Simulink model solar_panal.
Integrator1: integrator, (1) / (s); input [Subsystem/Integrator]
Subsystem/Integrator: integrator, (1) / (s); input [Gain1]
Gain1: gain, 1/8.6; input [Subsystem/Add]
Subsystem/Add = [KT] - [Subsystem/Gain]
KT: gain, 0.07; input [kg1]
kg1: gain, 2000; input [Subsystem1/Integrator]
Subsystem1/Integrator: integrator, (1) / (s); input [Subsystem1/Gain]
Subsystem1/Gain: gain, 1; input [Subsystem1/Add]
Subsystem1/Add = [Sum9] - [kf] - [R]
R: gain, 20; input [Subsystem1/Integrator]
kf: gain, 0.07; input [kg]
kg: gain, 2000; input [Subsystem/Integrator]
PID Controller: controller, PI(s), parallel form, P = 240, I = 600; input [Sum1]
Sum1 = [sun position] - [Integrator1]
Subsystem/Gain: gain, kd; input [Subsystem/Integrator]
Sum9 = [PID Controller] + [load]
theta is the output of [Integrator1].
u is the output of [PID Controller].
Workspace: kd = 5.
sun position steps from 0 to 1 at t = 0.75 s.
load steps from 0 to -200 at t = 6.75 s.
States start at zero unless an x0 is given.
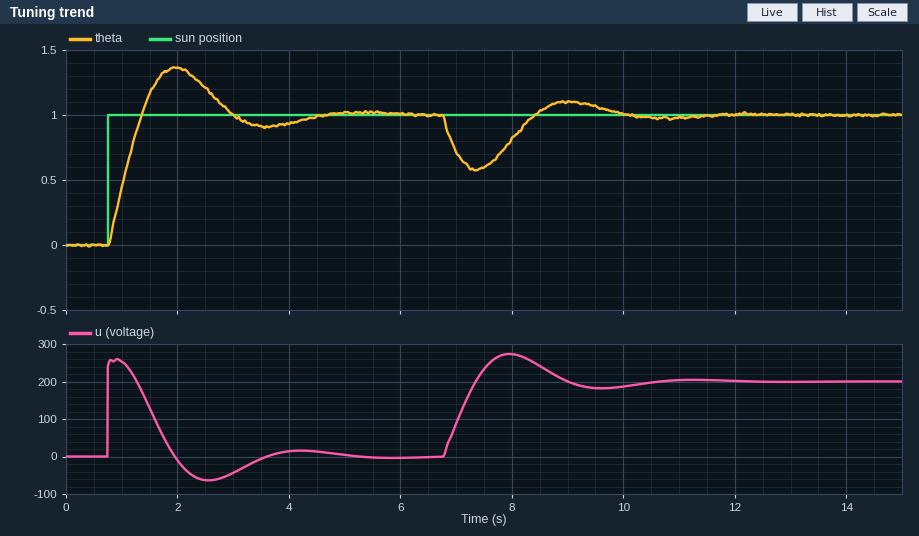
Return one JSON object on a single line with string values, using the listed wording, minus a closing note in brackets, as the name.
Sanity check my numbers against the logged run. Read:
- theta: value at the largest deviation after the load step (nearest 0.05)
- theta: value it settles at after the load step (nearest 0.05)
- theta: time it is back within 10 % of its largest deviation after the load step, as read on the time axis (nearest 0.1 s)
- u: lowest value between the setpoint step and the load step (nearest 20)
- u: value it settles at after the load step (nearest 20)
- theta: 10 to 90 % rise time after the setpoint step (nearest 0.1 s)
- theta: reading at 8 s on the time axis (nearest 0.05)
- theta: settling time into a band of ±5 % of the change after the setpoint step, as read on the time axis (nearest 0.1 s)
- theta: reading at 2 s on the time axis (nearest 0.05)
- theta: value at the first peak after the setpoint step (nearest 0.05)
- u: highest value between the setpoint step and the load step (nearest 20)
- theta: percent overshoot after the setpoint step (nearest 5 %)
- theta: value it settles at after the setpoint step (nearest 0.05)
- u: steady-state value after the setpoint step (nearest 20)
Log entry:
{"theta: value at the largest deviation after the load step": "0.60", "theta: value it settles at after the load step": "1.00", "theta: time it is back within 10 % of its largest deviation after the load step, as read on the time axis": "9.7 s", "u: lowest value between the setpoint step and the load step": "-60", "u: value it settles at after the load step": "200", "theta: 10 to 90 % rise time after the setpoint step": "0.5 s", "theta: reading at 8 s on the time axis": "0.80", "theta: settling time into a band of ±5 % of the change after the setpoint step, as read on the time axis": "4.2 s", "theta: reading at 2 s on the time axis": "1.35", "theta: value at the first peak after the setpoint step": "1.35", "u: highest value between the setpoint step and the load step": "260", "theta: percent overshoot after the setpoint step": "35 %", "theta: value it settles at after the setpoint step": "1.00", "u: steady-state value after the setpoint step": "0"}
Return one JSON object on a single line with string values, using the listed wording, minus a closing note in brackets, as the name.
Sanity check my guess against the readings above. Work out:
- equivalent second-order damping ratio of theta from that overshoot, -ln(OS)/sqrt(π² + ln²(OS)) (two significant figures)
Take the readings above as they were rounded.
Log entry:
{"equivalent second-order damping ratio of theta from that overshoot, -ln(OS)/sqrt(π² + ln²(OS))": "0.32"}
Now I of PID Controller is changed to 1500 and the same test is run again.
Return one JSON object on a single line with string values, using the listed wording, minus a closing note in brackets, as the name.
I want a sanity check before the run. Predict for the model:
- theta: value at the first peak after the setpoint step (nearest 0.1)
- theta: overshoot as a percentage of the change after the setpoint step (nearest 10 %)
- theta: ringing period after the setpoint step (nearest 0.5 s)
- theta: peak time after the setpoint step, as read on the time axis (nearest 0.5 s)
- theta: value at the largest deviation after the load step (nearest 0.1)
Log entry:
{"theta: value at the first peak after the setpoint step": "1.5", "theta: overshoot as a percentage of the change after the setpoint step": "50 %", "theta: ringing period after the setpoint step": "2.0 s", "theta: peak time after the setpoint step, as read on the time axis": "1.5 s", "theta: value at the largest deviation after the load step": "0.7"}
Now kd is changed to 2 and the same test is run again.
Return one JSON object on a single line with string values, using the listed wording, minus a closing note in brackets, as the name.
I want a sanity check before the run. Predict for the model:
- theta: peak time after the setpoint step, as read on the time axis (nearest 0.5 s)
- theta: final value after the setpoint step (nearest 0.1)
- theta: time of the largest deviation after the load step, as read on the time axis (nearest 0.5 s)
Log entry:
{"theta: peak time after the setpoint step, as read on the time axis": "2.0 s", "theta: final value after the setpoint step": "1.0", "theta: time of the largest deviation after the load step, as read on the time axis": "7.5 s"}
